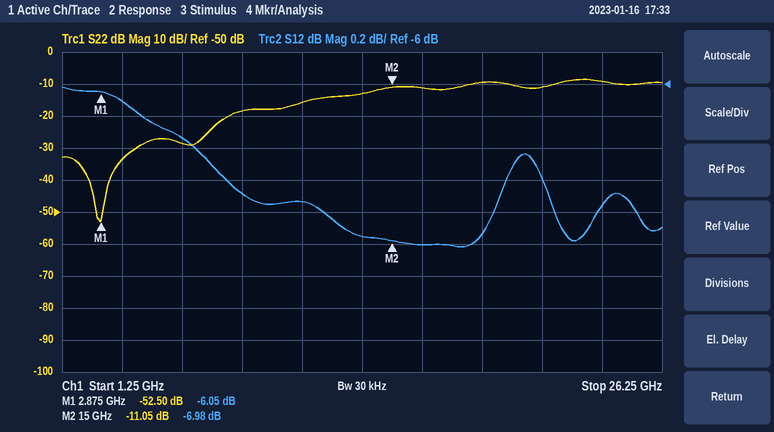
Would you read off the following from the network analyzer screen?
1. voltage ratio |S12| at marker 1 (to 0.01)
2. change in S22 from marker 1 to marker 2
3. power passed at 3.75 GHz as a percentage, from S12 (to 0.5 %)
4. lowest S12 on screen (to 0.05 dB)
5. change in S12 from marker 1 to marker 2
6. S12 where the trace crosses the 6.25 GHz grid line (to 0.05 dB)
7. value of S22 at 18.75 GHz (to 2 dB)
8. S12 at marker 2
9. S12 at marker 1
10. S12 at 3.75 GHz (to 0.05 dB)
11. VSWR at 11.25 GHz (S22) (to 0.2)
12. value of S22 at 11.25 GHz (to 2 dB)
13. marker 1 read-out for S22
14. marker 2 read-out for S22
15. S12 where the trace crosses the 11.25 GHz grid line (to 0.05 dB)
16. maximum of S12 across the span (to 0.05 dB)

0.50
41.45 dB
24.5 %
-7.00 dB
-0.93 dB
-6.35 dB
-10 dB
-6.98 dB
-6.05 dB
-6.10 dB
1.4
-16 dB
-52.50 dB
-11.05 dB
-6.75 dB
-6.00 dB
